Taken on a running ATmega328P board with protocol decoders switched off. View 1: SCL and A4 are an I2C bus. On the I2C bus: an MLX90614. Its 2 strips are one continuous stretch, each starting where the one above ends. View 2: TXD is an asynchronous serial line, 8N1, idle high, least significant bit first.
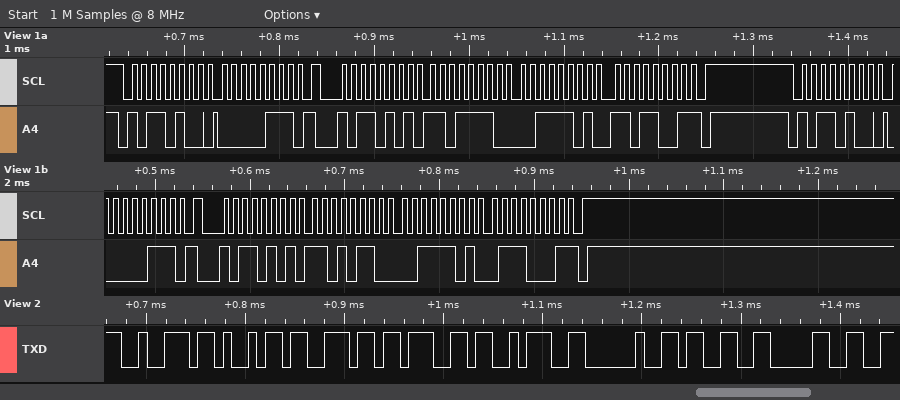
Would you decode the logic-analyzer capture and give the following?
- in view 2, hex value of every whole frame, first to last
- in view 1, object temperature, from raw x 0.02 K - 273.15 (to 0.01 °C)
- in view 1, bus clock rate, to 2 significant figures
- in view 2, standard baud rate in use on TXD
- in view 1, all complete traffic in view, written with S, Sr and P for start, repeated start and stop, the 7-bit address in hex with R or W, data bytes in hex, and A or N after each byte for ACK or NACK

72 69 6E 67 3A 20 33 30
43.61 °C
100 kHz
115200 baud
S 5AW A 07 A Sr 5AR A DE A 3D A D9 N P S 5AW A 07 A Sr 5AR A D6 A 3D A 71 N P
